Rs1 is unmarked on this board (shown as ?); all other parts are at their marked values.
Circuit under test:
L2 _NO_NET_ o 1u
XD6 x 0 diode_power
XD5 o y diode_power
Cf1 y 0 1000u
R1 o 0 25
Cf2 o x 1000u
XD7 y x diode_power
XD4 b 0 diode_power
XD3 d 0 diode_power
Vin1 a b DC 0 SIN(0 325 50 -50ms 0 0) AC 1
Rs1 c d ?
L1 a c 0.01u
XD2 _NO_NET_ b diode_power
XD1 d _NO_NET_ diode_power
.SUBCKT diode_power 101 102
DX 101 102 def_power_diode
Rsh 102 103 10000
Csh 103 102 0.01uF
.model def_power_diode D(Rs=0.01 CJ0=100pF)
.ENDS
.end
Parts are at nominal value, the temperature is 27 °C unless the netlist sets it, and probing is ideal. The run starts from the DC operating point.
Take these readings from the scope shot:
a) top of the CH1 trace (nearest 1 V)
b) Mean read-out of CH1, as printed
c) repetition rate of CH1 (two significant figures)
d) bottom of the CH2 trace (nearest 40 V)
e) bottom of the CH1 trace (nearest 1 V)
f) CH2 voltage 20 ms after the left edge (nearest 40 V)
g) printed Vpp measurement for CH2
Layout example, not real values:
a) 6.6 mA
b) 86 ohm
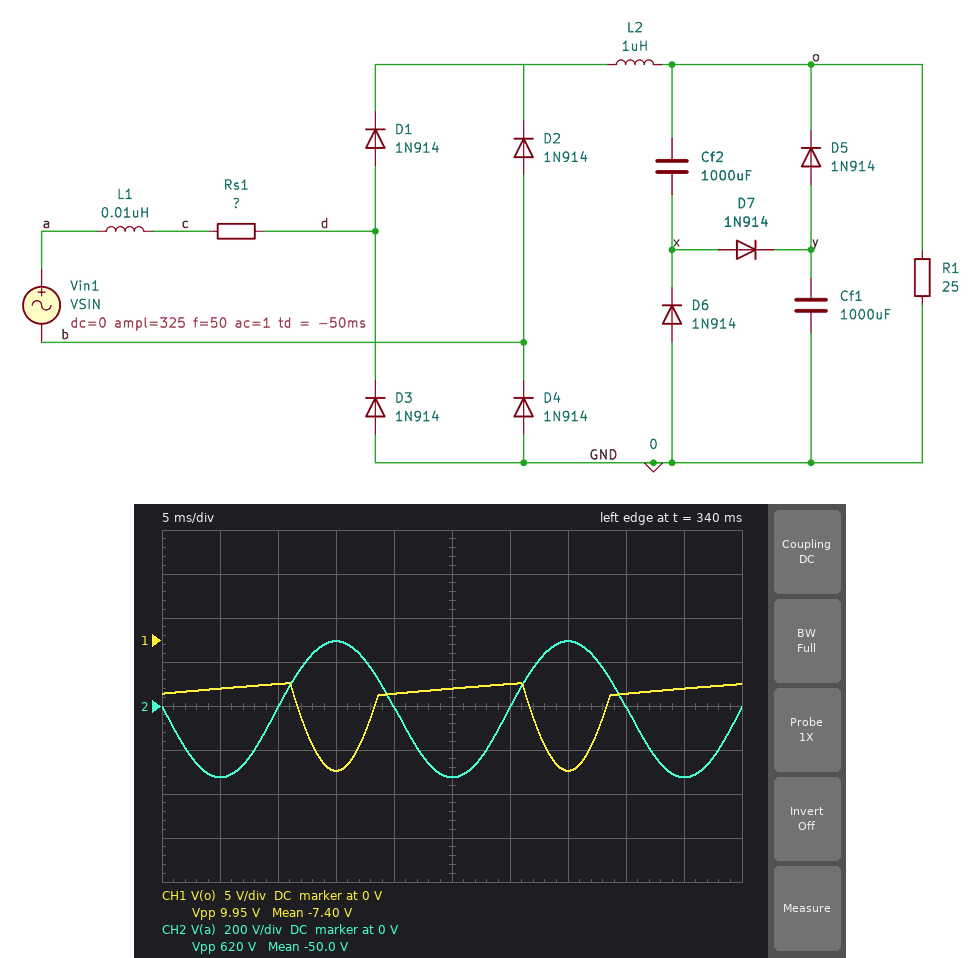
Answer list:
a) -5 V
b) -7.40 V
c) 50 Hz
d) -320 V
e) -15 V
f) 0 V
g) 620 V
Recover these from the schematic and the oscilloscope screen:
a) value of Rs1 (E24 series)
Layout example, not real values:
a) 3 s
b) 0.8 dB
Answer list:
a) 0.2 Ω
